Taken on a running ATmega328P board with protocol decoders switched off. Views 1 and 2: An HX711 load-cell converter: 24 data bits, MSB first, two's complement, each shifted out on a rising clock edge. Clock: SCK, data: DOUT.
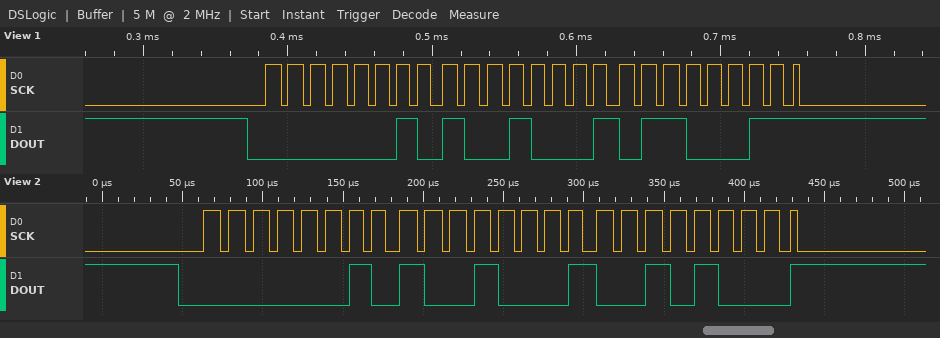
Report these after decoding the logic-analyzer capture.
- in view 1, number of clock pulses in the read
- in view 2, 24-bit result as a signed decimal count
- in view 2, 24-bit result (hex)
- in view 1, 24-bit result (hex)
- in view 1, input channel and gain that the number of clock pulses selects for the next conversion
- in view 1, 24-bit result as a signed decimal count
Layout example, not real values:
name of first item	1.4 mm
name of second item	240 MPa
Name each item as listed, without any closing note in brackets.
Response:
in view 1, number of clock pulses in the read	25
in view 2, 24-bit result as a signed decimal count	168232
in view 2, 24-bit result	0x029128
in view 1, 24-bit result	0x029163
in view 1, input channel and gain that the number of clock pulses selects for the next conversion	channel A, gain 128
in view 1, 24-bit result as a signed decimal count	168291
